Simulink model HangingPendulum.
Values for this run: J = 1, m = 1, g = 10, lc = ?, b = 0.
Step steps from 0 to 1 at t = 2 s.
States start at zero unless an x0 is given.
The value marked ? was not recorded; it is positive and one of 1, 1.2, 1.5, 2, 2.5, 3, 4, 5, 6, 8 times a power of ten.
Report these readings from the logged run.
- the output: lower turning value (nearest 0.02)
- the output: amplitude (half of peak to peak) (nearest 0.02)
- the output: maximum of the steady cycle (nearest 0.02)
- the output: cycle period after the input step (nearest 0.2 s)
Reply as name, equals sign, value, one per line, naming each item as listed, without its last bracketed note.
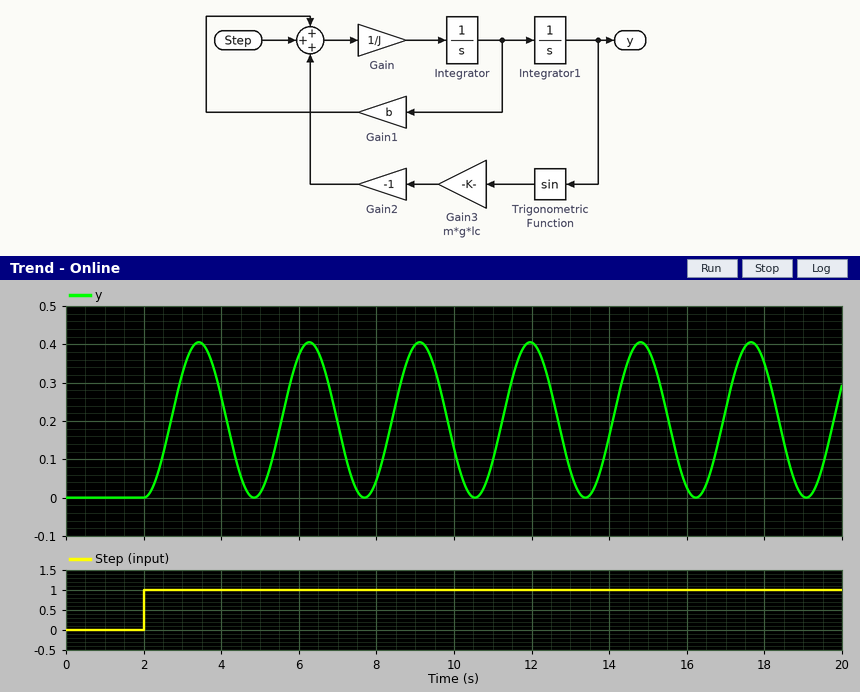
the output: lower turning value = 0.00
the output: amplitude (half of peak to peak) = 0.20
the output: maximum of the steady cycle = 0.40
the output: cycle period after the input step = 2.8 s
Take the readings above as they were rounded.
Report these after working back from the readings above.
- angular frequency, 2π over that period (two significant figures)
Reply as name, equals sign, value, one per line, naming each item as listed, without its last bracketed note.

angular frequency, 2π over that period = 2.2 rad/s
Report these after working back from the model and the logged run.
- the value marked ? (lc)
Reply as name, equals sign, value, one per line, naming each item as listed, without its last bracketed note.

the value marked ? = 0.5
